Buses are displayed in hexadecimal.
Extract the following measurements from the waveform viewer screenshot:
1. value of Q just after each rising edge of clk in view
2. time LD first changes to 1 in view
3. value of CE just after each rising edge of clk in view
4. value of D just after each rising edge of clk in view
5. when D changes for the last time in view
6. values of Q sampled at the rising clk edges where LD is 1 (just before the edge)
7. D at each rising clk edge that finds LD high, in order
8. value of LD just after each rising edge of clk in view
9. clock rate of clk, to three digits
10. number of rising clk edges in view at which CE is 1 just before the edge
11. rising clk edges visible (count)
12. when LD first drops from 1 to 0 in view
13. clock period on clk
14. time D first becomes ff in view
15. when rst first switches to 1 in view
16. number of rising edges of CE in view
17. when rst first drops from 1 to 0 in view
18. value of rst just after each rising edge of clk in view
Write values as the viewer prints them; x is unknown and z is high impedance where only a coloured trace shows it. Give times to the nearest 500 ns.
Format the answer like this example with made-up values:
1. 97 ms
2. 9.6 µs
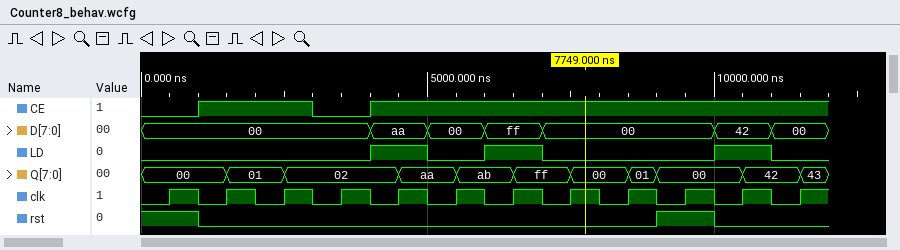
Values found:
1. 00, 01, 02, 02, aa, ab, ff, 00, 01, 00, 42, 43
2. 4000 ns
3. 0 1 1 0 1 1 1 1 1 1 1 1
4. 00, 00, 00, 00, aa, 00, ff, 00, 00, 00, 42, 00
5. 11000 ns
6. 02, ab, 00
7. aa, ff, 42
8. 0 0 0 0 1 0 1 0 0 0 1 0
9. 1.00 MHz
10. 10
11. 12
12. 5000 ns
13. 1000 ns
14. 6000 ns
15. 9000 ns
16. 2
17. 1000 ns
18. 1 0 0 0 0 0 0 0 0 1 0 0
